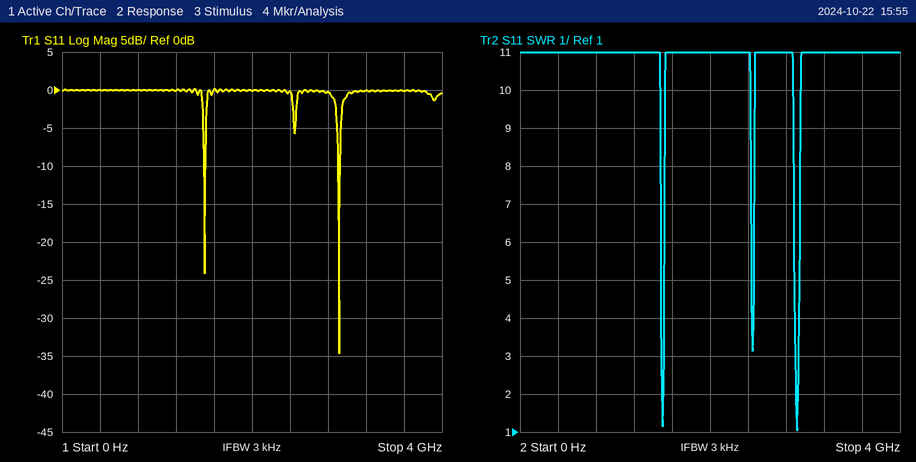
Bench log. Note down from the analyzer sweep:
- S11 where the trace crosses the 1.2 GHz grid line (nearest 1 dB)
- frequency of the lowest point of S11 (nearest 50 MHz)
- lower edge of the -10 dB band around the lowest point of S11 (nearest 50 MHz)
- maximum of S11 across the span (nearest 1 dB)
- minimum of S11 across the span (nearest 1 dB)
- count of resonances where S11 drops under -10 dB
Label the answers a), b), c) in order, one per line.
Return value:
a) 0 dB
b) 2.90 GHz
c) 2.90 GHz
d) 0 dB
e) -35 dB
f) 2
